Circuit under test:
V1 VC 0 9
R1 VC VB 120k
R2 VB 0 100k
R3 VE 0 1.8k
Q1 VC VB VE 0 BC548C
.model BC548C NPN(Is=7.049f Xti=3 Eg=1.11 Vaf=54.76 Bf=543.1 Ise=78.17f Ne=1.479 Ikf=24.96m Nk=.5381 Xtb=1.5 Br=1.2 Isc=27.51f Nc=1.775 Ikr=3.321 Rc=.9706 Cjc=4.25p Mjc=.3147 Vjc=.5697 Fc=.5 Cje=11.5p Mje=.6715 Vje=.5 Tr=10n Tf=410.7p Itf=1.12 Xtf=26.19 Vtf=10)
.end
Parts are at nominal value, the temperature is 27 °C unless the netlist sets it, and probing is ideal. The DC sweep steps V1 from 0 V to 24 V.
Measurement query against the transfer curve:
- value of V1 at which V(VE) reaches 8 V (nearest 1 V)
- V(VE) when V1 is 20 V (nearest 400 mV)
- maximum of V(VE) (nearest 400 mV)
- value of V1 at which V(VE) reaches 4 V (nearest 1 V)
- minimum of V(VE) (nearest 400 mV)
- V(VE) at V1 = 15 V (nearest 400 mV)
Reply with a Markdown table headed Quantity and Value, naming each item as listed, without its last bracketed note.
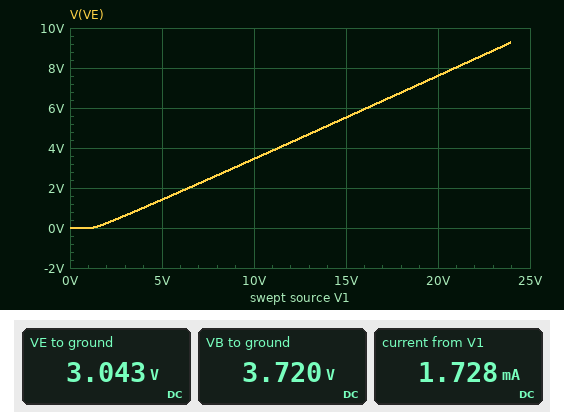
| Quantity | Value |
|---|---|
| value of V1 at which V(VE) reaches 8 V | 21 V |
| V(VE) when V1 is 20 V | 7.6 V |
| maximum of V(VE) | 9.2 V |
| value of V1 at which V(VE) reaches 4 V | 11 V |
| minimum of V(VE) | 0 V |
| V(VE) at V1 = 15 V | 5.6 V |
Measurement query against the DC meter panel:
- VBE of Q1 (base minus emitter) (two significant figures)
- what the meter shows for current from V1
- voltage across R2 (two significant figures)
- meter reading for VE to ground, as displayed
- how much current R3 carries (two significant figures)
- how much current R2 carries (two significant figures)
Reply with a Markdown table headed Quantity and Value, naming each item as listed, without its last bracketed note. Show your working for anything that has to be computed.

| Quantity | Value |
|---|---|
| VBE of Q1 (base minus emitter) | 3.72 V - 3.043 V = 680 mV |
| what the meter shows for current from V1 | 1.728 mA |
| voltage across R2 | 3.72 V = 3.7 V |
| meter reading for VE to ground, as displayed | 3.043 V |
| how much current R3 carries | (3.043 V) / 1.8 kΩ = 1.7 mA |
| how much current R2 carries | (3.72 V) / 100 kΩ = 37 µA |
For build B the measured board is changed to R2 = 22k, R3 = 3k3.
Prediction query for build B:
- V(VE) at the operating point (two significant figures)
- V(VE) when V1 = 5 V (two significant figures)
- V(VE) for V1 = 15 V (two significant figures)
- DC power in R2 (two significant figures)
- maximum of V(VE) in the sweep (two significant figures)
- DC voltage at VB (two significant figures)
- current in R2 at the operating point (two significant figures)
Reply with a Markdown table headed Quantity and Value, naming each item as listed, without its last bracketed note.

| Quantity | Value |
|---|---|
| V(VE) at the operating point | 750 mV |
| V(VE) when V1 = 5 V | 180 mV |
| V(VE) for V1 = 15 V | 1.6 V |
| DC power in R2 | 85 µW |
| maximum of V(VE) in the sweep | 3.0 V |
| DC voltage at VB | 1.4 V |
| current in R2 at the operating point | 62 µA |
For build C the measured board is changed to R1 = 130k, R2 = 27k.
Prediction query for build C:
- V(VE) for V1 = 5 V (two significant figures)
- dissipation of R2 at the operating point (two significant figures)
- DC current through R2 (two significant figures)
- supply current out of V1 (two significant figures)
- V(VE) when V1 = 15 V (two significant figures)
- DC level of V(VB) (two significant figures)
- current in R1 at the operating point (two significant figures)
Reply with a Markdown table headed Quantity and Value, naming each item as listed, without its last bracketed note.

| Quantity | Value |
|---|---|
| V(VE) for V1 = 5 V | 230 mV |
| dissipation of R2 at the operating point | 83 µW |
| DC current through R2 | 55 µA |
| supply current out of V1 | 530 µA |
| V(VE) when V1 = 15 V | 1.8 V |
| DC level of V(VB) | 1.5 V |
| current in R1 at the operating point | 58 µA |
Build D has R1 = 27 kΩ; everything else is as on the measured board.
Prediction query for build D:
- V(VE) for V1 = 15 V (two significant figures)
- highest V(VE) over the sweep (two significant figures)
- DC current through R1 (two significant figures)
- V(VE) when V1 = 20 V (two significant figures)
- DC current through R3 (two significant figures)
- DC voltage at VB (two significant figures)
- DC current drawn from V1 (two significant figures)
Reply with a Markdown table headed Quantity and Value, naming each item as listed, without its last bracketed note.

| Quantity | Value |
|---|---|
| V(VE) for V1 = 15 V | 11 V |
| highest V(VE) over the sweep | 17 V |
| DC current through R1 | 81 µA |
| V(VE) when V1 = 20 V | 14 V |
| DC current through R3 | 3.4 mA |
| DC voltage at VB | 6.8 V |
| DC current drawn from V1 | 3.5 mA |
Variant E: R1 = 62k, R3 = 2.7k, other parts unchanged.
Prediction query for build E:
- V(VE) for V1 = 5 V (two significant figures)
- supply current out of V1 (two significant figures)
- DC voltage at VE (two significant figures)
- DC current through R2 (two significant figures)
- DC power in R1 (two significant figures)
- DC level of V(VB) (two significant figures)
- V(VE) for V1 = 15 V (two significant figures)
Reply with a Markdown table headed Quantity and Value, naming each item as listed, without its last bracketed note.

| Quantity | Value |
|---|---|
| V(VE) for V1 = 5 V | 2.3 V |
| supply current out of V1 | 1.8 mA |
| DC voltage at VE | 4.6 V |
| DC current through R2 | 53 µA |
| DC power in R1 | 220 µW |
| DC level of V(VB) | 5.3 V |
| V(VE) for V1 = 15 V | 8.1 V |
